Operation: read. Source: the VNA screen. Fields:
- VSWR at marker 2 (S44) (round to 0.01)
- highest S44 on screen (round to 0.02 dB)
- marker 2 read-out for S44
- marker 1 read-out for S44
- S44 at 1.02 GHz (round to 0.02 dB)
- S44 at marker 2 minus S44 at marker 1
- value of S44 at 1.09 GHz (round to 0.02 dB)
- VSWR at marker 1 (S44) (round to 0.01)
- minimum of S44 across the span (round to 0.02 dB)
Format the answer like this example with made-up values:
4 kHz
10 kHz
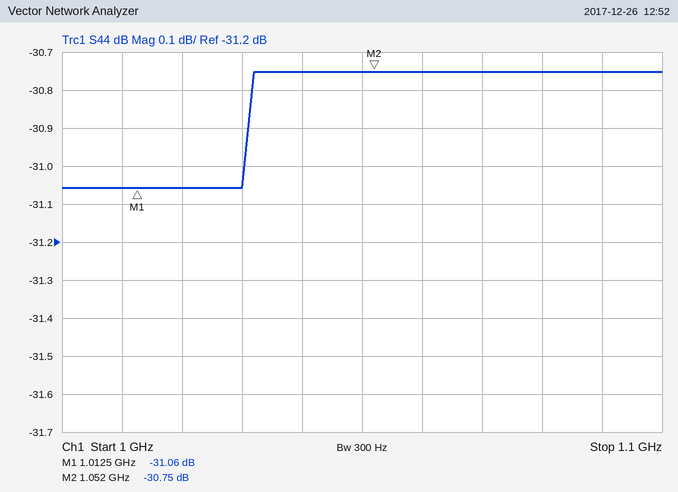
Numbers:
1.06
-30.76 dB
-30.75 dB
-31.06 dB
-31.06 dB
0.31 dB
-30.76 dB
1.06
-31.06 dB
